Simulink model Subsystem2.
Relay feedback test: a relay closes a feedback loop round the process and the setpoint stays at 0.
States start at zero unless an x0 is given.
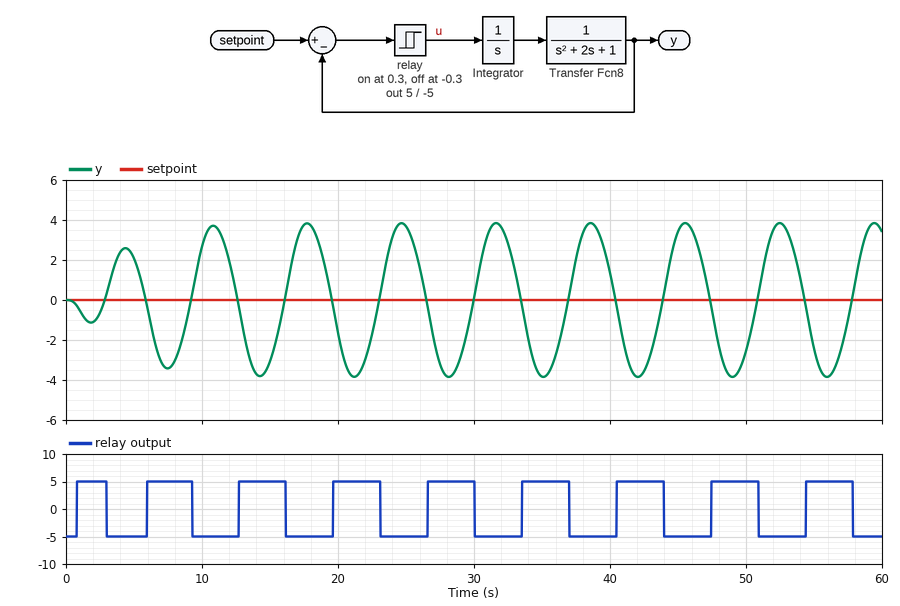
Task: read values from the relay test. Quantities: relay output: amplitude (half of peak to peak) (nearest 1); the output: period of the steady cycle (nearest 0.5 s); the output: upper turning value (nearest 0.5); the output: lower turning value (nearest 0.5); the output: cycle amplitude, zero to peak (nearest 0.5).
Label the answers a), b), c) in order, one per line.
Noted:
a) 5
b) 7.0 s
c) 4.0
d) -4.0
e) 4.0
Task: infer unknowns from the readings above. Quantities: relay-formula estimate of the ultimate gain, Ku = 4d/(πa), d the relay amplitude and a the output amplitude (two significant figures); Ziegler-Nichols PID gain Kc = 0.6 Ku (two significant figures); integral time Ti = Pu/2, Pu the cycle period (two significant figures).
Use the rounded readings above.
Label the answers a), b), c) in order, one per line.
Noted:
a) 1.6
b) 0.96
c) 3.5 s
